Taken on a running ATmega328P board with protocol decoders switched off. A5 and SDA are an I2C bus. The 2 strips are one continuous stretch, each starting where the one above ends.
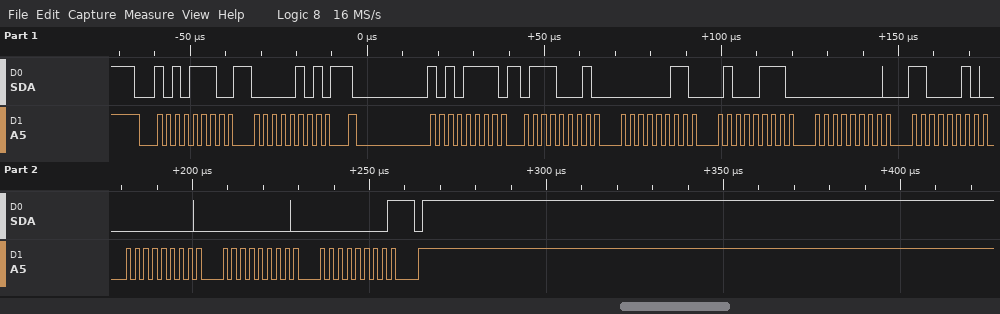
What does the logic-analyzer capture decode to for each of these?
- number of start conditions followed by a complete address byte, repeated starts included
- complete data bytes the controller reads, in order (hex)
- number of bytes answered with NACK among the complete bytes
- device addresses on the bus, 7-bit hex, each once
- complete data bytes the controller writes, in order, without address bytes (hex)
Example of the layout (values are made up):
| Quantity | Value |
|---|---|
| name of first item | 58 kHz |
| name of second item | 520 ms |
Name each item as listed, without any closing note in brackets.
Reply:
| Quantity | Value |
|---|---|
| number of start conditions followed by a complete address byte, repeated starts included | 2 |
| complete data bytes the controller reads, in order | 71 03 47 00 C2 00 00 00 |
| number of bytes answered with NACK among the complete bytes | 1 |
| device addresses on the bus, 7-bit hex, each once | 0x57 |
| complete data bytes the controller writes, in order, without address bytes | 05 |
